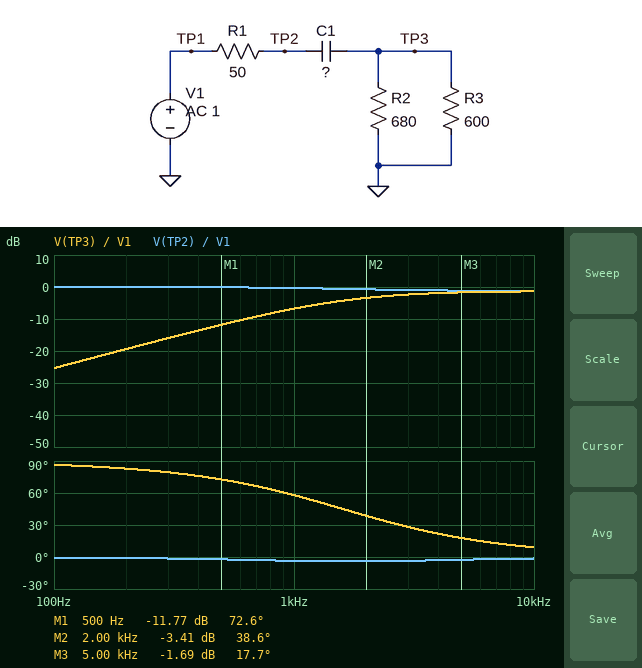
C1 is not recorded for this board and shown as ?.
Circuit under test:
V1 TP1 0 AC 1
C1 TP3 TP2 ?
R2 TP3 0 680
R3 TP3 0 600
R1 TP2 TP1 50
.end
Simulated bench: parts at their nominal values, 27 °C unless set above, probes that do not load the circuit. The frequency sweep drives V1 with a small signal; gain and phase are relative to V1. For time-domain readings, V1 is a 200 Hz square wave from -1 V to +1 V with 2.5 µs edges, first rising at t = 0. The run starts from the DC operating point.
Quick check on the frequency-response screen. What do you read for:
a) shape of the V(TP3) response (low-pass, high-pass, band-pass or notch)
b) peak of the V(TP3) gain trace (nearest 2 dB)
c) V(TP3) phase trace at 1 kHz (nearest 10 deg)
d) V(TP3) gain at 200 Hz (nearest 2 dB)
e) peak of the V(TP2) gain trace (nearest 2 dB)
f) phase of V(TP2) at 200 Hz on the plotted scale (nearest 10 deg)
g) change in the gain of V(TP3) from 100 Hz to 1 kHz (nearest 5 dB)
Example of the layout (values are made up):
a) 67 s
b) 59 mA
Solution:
a) high-pass
b) -2 dB
c) 60 deg
d) -20 dB
e) 0 dB
f) 0 deg
g) 20 dB
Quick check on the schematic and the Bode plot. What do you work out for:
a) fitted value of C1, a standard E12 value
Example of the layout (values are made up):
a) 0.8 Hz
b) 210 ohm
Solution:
a) 270 nF
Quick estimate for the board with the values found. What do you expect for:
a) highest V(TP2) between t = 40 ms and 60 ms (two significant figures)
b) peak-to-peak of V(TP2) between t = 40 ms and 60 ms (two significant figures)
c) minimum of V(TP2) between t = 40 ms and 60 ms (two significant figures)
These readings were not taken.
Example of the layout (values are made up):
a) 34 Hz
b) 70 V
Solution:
a) 1.0 V
b) 2.0 V
c) -1.0 V
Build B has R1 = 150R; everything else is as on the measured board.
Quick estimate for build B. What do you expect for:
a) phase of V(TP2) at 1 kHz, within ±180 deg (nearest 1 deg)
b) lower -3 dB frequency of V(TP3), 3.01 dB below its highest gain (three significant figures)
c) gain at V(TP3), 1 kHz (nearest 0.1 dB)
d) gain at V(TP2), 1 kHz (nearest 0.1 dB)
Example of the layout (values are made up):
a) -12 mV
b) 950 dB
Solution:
a) -10 deg
b) 1.26 kHz
c) -7.5 dB
d) -1.0 dB
